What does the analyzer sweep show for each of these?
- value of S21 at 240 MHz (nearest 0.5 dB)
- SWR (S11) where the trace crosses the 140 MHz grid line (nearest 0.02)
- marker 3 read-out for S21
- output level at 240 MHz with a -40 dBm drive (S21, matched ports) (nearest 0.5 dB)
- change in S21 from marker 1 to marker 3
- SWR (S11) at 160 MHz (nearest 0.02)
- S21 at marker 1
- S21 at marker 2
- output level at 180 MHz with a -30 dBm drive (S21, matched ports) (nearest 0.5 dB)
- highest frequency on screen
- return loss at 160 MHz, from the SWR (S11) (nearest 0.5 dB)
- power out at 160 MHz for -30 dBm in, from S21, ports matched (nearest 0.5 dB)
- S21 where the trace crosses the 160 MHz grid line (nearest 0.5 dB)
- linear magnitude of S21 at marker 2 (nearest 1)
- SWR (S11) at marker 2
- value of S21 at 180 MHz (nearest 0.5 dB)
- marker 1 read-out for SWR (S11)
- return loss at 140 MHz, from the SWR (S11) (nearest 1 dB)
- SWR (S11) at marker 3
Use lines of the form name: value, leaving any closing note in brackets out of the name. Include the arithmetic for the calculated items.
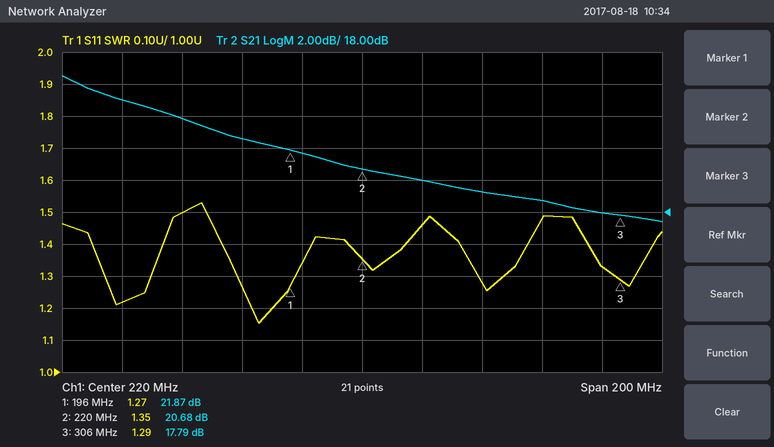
value of S21 at 240 MHz: 20.0 dB
SWR (S11) where the trace crosses the 140 MHz grid line: 1.22
marker 3 read-out for S21: 17.79 dB
output level at 240 MHz with a -40 dBm drive (S21, matched ports): -40 dBm + (20.0 dB) = -20.0 dBm
change in S21 from marker 1 to marker 3: 17.79 − (21.87) = -4.08 dB
SWR (S11) at 160 MHz: 1.50
S21 at marker 1: 21.87 dB
S21 at marker 2: 20.68 dB
output level at 180 MHz with a -30 dBm drive (S21, matched ports): -30 dBm + (22.5 dB) = -7.5 dBm
highest frequency on screen: 320 MHz
return loss at 160 MHz, from the SWR (S11): −20 log10((1.5 − 1)/(1.5 + 1)) ≈ 14.0 dB
power out at 160 MHz for -30 dBm in, from S21, ports matched: -30 dBm + (24.0 dB) = -6.0 dBm
S21 where the trace crosses the 160 MHz grid line: 24.0 dB
linear magnitude of S21 at marker 2: 10^(20.68/20) ≈ 11
SWR (S11) at marker 2: 1.35
value of S21 at 180 MHz: 22.5 dB
marker 1 read-out for SWR: 1.27
return loss at 140 MHz, from the SWR (S11): −20 log10((1.22 − 1)/(1.22 + 1)) ≈ 20 dB
SWR (S11) at marker 3: 1.29
